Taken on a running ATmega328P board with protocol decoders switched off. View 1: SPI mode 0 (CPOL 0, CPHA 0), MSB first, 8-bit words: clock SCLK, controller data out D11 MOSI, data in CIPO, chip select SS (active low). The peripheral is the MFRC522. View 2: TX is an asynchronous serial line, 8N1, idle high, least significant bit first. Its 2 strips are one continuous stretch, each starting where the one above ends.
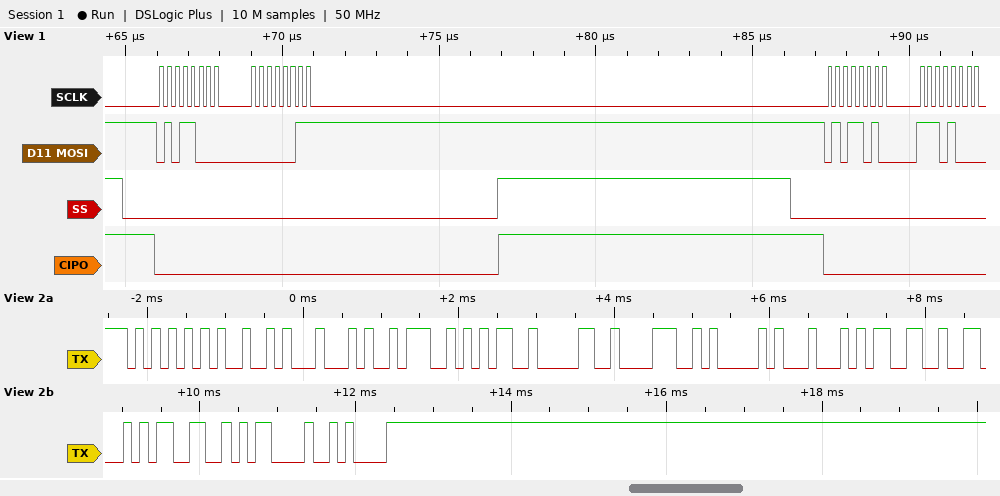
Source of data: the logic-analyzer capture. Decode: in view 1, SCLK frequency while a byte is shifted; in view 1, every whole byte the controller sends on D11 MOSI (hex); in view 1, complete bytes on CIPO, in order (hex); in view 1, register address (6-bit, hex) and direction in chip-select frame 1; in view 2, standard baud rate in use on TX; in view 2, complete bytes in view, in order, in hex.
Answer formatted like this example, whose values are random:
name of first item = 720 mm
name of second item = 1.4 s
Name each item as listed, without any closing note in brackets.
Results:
in view 1, SCLK frequency while a byte is shifted = 4 MHz
in view 1, every whole byte the controller sends on D11 MOSI = 58 03 5A E8
in view 1, complete bytes on CIPO, in order = 00 00 00 00
in view 1, register address (6-bit, hex) and direction in chip-select frame 1 = 0x2C write
in view 2, standard baud rate in use on TX = 9600 baud
in view 2, complete bytes in view, in order, in hex = 0x55 0x49 0x44 0x3A 0x35 0x30 0x38 0x41 0x44 0x33 0x46 0x33 0x0D 0x0A
